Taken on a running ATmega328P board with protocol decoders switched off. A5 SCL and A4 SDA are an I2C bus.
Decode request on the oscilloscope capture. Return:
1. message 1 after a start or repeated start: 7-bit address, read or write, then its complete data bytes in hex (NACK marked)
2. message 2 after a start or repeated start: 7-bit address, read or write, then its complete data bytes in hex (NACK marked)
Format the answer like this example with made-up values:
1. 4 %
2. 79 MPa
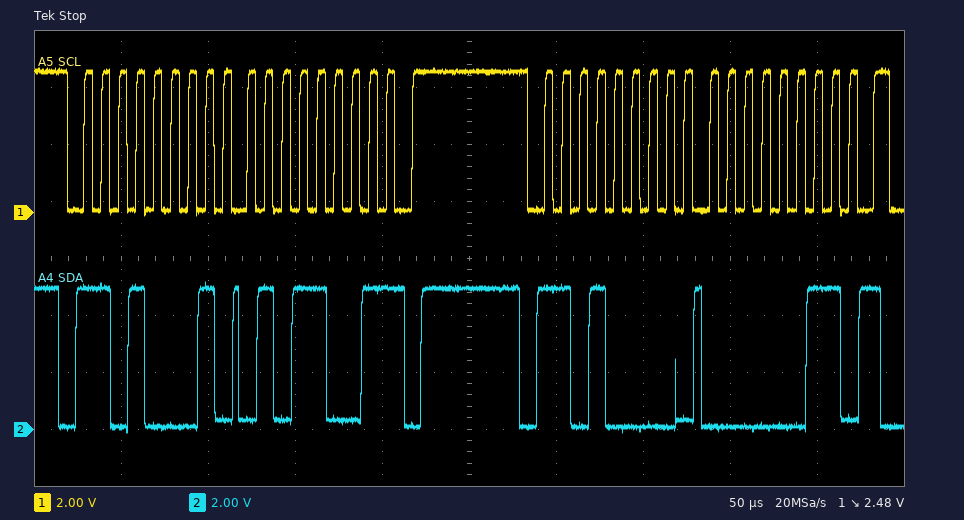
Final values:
1. 0x68 read: 59 NACK
2. 0x68 write: 03
